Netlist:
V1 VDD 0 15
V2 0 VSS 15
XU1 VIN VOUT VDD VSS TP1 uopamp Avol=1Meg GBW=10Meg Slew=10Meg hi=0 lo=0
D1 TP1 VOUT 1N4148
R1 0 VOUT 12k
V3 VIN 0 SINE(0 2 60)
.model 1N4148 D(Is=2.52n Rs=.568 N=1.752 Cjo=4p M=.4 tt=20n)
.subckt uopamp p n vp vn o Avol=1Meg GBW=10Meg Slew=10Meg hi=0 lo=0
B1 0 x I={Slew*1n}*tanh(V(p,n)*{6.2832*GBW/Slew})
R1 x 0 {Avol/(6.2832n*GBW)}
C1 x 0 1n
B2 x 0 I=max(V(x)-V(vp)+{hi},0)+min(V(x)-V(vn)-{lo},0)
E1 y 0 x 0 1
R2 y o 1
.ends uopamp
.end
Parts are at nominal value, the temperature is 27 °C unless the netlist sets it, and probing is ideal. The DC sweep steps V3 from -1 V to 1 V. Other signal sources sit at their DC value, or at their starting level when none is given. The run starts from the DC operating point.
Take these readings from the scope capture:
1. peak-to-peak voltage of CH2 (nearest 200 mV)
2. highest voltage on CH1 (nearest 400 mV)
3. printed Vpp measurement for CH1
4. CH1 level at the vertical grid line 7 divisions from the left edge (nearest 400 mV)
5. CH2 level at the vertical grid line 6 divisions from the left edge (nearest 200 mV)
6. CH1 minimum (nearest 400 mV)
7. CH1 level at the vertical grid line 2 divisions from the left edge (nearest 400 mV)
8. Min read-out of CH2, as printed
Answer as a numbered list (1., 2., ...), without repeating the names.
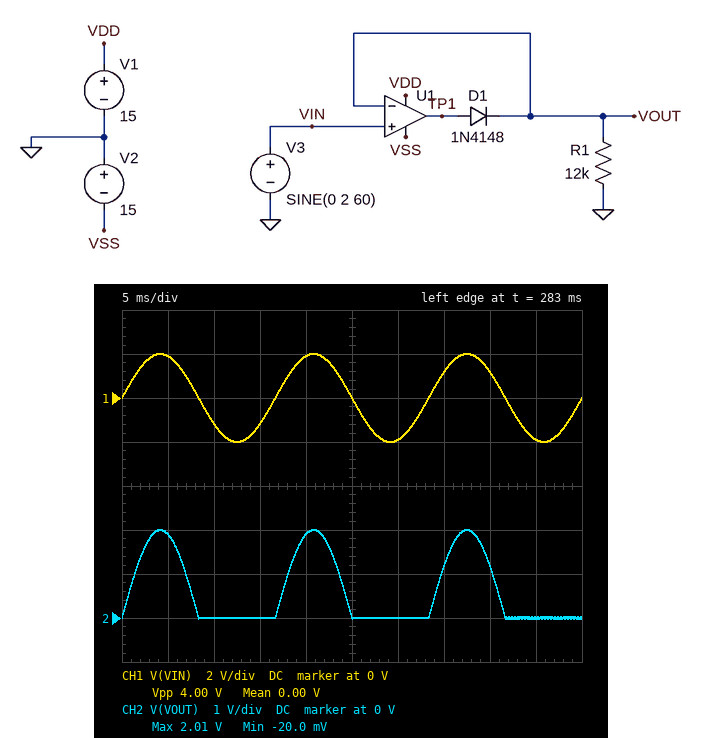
1. 2.0 V
2. 2.0 V
3. 4.00 V
4. 1.2 V
5. 0 V
6. -2.0 V
7. -1.2 V
8. -20.0 mV
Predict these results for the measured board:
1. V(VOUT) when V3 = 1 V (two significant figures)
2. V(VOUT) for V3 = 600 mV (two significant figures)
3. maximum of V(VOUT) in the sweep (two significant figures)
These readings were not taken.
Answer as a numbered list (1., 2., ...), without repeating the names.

1. 1.0 V
2. 600 mV
3. 1.0 V
